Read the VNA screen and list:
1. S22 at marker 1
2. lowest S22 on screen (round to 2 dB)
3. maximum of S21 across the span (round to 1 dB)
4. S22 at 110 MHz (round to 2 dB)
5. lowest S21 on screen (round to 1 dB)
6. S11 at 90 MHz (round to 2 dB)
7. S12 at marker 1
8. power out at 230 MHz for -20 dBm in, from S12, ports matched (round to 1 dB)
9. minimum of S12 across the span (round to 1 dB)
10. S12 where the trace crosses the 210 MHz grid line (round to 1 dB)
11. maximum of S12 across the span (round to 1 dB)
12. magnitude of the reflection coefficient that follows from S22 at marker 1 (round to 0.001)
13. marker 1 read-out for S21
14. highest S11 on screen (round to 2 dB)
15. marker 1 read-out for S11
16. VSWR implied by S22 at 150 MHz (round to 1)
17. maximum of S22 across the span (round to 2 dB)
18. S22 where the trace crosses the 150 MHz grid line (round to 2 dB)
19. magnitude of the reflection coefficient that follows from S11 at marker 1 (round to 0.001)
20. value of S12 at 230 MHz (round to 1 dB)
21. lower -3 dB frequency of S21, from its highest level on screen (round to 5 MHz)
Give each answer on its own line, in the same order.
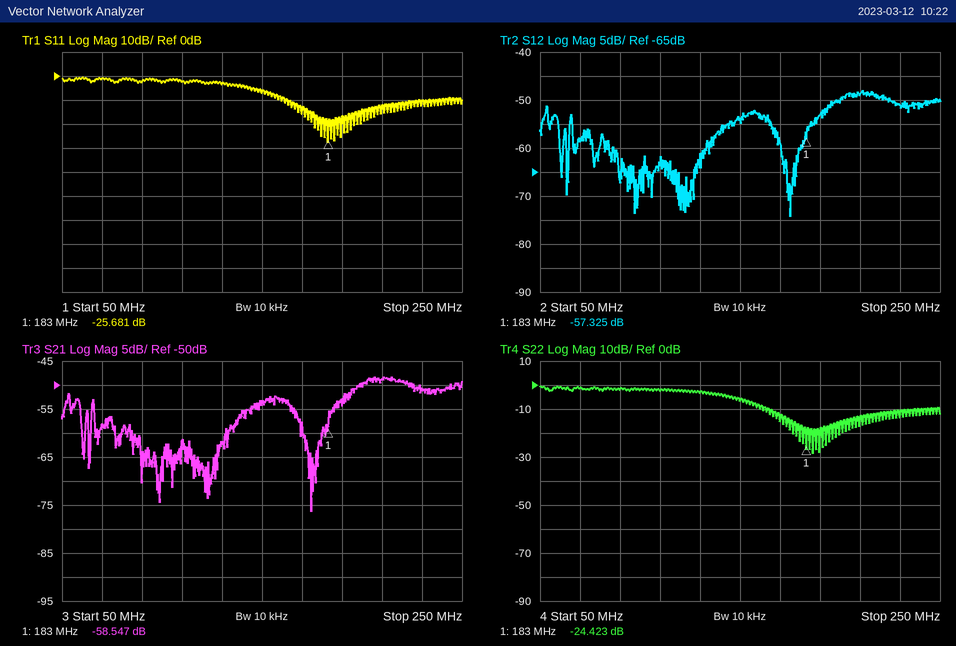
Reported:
-24.423 dB
-28 dB
-48 dB
-2 dB
-76 dB
-2 dB
-57.325 dB
-71 dBm
-74 dB
-49 dB
-48 dB
0.060
-58.547 dB
0 dB
-25.681 dB
3
0 dB
-6 dB
0.052
-51 dB
195 MHz
